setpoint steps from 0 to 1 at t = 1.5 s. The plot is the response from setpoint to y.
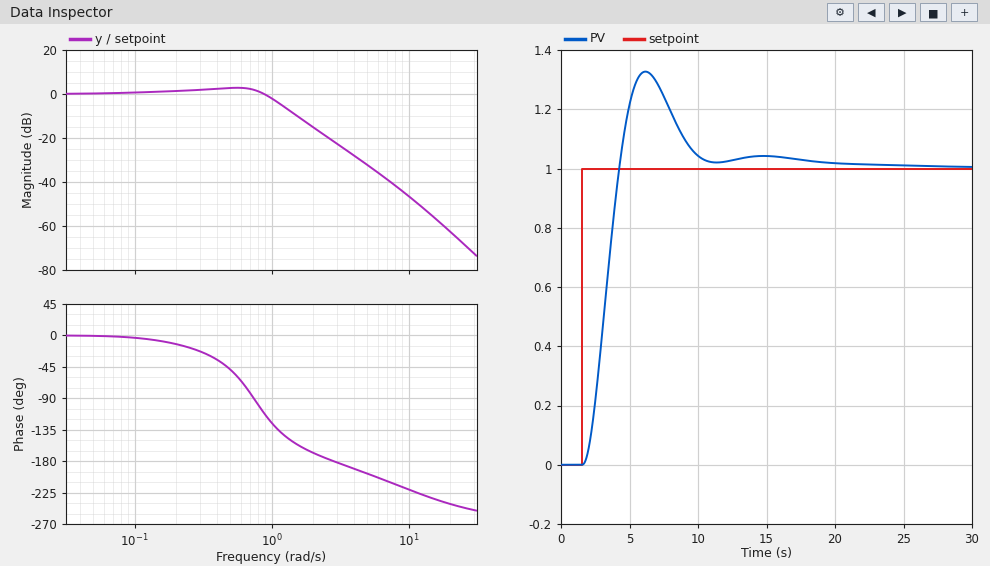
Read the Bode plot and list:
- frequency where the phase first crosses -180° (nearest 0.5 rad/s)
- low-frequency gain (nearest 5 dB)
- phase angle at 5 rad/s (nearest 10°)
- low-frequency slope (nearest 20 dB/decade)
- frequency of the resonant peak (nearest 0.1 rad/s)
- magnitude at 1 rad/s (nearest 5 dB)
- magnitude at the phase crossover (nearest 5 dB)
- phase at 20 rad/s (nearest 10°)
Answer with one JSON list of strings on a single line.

["3.0 rad/s", "0 dB", "-200°", "0 dB/decade", "0.5 rad/s", "0 dB", "-20 dB", "-240°"]
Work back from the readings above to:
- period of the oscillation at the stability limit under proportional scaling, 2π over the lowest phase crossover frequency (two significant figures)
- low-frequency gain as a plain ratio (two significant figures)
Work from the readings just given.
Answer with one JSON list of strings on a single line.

["2.1 s", "1.0"]
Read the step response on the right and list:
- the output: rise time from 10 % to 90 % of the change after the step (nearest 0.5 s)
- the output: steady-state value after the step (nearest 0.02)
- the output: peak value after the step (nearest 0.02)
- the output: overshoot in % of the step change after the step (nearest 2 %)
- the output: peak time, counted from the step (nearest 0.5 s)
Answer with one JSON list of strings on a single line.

["2.0 s", "1.00", "1.32", "32 %", "4.5 s"]
